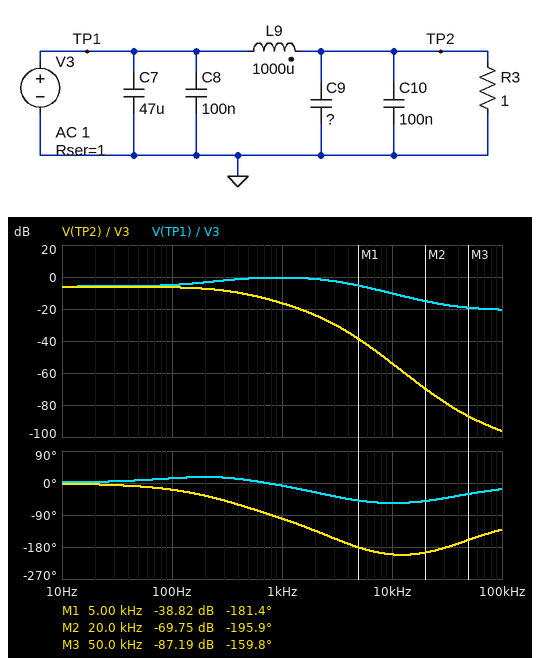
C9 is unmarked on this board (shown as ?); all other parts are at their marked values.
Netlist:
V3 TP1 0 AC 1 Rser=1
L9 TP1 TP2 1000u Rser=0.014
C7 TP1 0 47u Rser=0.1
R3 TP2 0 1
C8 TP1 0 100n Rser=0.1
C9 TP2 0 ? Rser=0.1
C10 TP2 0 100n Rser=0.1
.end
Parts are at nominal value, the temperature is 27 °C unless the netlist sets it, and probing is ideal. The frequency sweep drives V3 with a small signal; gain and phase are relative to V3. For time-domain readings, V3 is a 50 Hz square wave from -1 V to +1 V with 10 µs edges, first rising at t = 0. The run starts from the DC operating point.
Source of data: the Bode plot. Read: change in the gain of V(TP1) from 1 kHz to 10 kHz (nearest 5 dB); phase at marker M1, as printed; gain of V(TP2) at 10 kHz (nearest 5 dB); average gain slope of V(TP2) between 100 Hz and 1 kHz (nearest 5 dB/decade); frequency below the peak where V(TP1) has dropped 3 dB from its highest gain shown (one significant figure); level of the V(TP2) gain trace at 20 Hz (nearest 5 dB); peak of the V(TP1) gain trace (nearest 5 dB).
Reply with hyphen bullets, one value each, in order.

- -10 dB
- -181.4 deg
- -55 dB
- -10 dB/decade
- 200 Hz
- -5 dB
- 0 dB
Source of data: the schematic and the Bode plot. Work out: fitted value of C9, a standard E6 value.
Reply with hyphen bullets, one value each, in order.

- 33 µF
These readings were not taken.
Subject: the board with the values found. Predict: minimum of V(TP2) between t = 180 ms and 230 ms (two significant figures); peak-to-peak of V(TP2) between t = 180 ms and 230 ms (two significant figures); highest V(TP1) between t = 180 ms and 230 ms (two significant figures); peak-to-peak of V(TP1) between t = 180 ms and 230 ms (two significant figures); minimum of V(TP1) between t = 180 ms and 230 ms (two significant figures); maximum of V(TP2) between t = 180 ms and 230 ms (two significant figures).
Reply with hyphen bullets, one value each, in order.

- -500 mV
- 990 mV
- 1.3 V
- 2.6 V
- -1.3 V
- 500 mV
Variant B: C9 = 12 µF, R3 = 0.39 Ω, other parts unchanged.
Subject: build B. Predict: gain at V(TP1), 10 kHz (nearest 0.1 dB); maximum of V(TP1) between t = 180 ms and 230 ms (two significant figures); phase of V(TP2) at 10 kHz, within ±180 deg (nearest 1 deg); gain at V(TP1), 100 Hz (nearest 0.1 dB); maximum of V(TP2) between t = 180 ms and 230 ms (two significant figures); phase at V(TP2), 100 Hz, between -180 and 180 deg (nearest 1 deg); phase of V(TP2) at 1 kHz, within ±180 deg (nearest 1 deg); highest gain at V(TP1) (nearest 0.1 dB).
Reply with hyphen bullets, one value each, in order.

- -10.2 dB
- 1.5 V
- -162 deg
- -6.2 dB
- 280 mV
- -25 deg
- -96 deg
- -0.2 dB
